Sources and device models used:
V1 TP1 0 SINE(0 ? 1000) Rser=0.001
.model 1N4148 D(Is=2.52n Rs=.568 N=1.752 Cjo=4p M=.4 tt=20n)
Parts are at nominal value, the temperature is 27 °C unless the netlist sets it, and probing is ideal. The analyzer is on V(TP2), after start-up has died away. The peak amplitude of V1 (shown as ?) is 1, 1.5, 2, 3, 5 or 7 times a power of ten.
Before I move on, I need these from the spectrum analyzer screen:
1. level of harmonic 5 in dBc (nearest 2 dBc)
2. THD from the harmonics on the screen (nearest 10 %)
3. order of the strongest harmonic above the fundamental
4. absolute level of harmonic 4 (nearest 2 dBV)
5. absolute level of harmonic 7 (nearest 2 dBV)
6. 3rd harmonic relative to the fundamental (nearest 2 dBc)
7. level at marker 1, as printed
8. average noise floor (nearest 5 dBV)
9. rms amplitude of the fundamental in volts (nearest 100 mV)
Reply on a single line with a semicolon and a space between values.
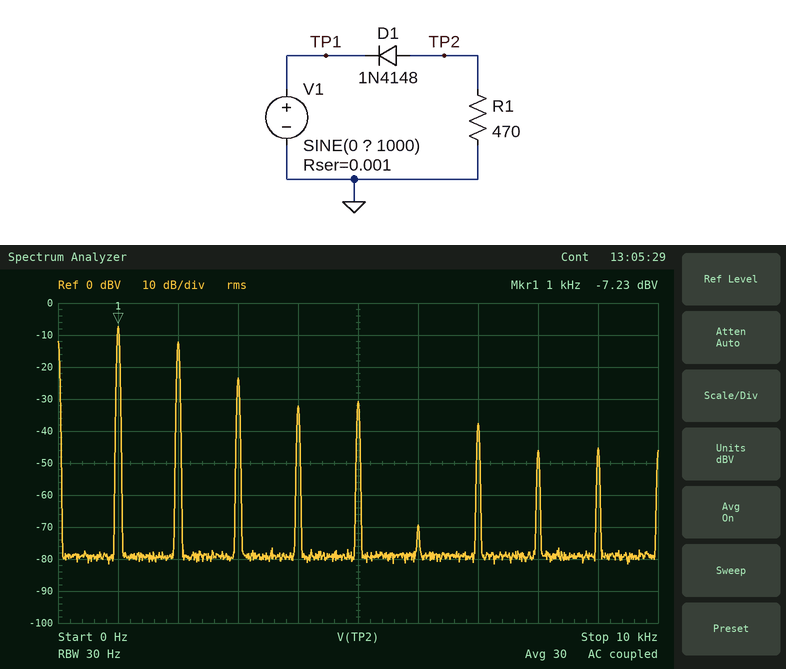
-24 dBc; 60 %; 2; -32 dBV; -38 dBV; -16 dBc; -7.23 dBV; -80 dBV; 400 mV
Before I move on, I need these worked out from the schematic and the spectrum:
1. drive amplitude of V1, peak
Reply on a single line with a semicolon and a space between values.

2 V
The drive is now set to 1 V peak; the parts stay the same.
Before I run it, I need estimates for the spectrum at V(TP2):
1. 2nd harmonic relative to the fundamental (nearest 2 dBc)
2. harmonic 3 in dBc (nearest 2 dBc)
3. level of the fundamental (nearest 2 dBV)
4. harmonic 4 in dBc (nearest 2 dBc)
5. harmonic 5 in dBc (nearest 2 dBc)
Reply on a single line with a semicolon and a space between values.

-4 dBc; -10 dBc; -18 dBV; -24 dBc; -26 dBc
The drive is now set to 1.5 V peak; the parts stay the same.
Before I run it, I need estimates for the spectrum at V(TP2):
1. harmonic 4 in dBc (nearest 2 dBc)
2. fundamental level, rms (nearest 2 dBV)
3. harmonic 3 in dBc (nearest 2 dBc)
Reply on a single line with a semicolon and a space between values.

-32 dBc; -12 dBV; -14 dBc
